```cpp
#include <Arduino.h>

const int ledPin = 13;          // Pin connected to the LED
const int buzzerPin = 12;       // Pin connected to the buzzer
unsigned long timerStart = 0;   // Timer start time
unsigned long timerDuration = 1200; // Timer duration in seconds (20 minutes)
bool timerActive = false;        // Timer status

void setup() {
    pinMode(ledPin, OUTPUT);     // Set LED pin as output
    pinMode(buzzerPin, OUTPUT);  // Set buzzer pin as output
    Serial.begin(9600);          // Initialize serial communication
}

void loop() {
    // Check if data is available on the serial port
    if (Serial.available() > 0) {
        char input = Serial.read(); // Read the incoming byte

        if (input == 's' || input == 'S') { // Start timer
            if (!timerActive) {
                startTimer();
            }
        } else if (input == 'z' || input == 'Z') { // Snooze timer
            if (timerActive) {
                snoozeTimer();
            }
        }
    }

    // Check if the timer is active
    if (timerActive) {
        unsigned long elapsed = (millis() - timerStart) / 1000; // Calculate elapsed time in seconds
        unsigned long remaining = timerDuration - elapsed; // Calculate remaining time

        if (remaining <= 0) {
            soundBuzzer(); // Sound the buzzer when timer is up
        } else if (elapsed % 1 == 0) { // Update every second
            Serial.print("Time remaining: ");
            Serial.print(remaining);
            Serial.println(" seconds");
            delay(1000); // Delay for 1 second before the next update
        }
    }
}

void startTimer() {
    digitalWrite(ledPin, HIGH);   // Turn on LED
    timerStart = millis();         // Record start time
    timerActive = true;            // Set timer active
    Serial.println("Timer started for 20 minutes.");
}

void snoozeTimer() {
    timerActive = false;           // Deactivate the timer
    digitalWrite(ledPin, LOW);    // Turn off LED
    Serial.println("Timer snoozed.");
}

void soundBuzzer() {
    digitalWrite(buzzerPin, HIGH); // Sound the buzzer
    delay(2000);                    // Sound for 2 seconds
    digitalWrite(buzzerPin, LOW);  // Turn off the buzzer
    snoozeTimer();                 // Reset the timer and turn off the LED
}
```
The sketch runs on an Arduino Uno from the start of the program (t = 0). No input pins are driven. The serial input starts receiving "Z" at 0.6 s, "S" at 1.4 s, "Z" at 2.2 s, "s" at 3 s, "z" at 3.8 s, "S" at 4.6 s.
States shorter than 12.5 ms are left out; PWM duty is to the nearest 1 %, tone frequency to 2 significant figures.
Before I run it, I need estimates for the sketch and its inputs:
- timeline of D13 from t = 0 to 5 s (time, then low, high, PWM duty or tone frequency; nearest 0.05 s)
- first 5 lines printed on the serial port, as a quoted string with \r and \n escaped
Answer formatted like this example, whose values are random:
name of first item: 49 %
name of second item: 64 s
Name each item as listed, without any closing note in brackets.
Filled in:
timeline of D13 from t = 0 to 5 s: 0 s low; 1.4 s high; 2.4 s low; 3 s high; 4 s low; 4.6 s high
first 5 lines printed on the serial port, as a quoted string with \r and \n escaped: "Timer started for 20 minutes.\r\nTime remaining: 1200 seconds\r\nTimer snoozed.\r\nTimer started for 20 minutes.\r\nTime remaining: 1200 seconds\r\n"
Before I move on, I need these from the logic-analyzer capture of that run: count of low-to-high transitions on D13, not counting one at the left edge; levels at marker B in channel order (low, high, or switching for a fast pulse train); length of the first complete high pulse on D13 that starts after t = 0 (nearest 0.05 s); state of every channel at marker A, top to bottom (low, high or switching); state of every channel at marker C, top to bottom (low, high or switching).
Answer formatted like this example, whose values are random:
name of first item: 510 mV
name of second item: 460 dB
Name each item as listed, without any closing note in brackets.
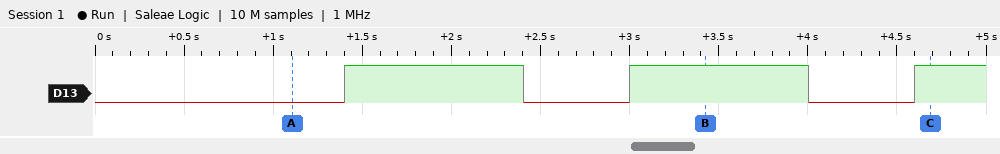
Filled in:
count of low-to-high transitions on D13, not counting one at the left edge: 3
levels at marker B in channel order: D13 high
length of the first complete high pulse on D13 that starts after t = 0: 1.00 s
state of every channel at marker A, top to bottom: D13 low
state of every channel at marker C, top to bottom: D13 high
